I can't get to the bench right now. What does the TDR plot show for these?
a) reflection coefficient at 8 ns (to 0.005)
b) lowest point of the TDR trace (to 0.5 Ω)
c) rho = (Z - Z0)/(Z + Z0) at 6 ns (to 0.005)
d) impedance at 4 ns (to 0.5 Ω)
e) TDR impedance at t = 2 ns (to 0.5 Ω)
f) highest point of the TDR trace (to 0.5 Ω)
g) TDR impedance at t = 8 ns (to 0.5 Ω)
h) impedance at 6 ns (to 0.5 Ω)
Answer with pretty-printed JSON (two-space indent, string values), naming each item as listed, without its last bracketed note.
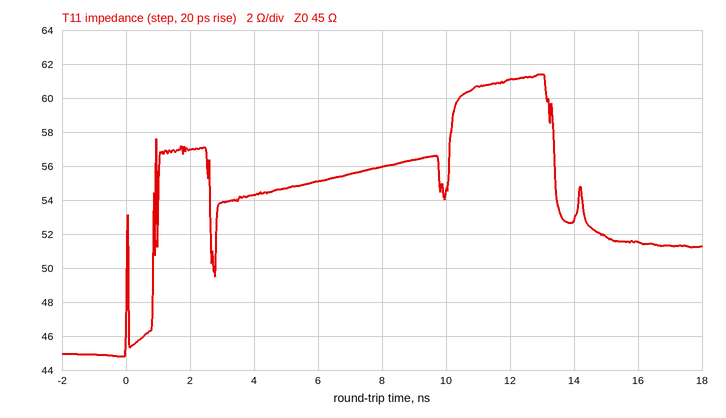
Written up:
{
  "reflection coefficient at 8 ns": "+0.110",
  "lowest point of the TDR trace": "45.0 Ω",
  "rho = (Z - Z0)/(Z + Z0) at 6 ns": "+0.100",
  "impedance at 4 ns": "54.5 Ω",
  "TDR impedance at t = 2 ns": "57.0 Ω",
  "highest point of the TDR trace": "61.5 Ω",
  "TDR impedance at t = 8 ns": "56.0 Ω",
  "impedance at 6 ns": "55.0 Ω"
}
